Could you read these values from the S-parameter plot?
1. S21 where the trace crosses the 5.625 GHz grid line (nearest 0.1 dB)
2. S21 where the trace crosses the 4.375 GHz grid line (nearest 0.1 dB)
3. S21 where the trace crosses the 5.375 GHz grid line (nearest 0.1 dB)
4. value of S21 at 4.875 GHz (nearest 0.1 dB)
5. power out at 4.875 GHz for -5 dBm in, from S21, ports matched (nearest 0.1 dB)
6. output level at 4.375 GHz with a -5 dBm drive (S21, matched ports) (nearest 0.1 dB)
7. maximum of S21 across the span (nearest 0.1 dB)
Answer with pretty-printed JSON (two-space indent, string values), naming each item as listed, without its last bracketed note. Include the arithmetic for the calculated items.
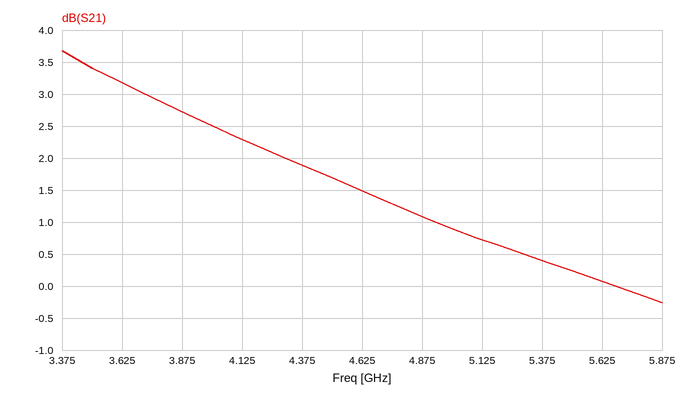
{
  "S21 where the trace crosses the 5.625 GHz grid line": "0.1 dB",
  "S21 where the trace crosses the 4.375 GHz grid line": "1.9 dB",
  "S21 where the trace crosses the 5.375 GHz grid line": "0.4 dB",
  "value of S21 at 4.875 GHz": "1.1 dB",
  "power out at 4.875 GHz for -5 dBm in, from S21, ports matched": "-5 dBm + (1.1 dB) = -3.9 dBm",
  "output level at 4.375 GHz with a -5 dBm drive (S21, matched ports)": "-5 dBm + (1.9 dB) = -3.1 dBm",
  "maximum of S21 across the span": "3.7 dB"
}
